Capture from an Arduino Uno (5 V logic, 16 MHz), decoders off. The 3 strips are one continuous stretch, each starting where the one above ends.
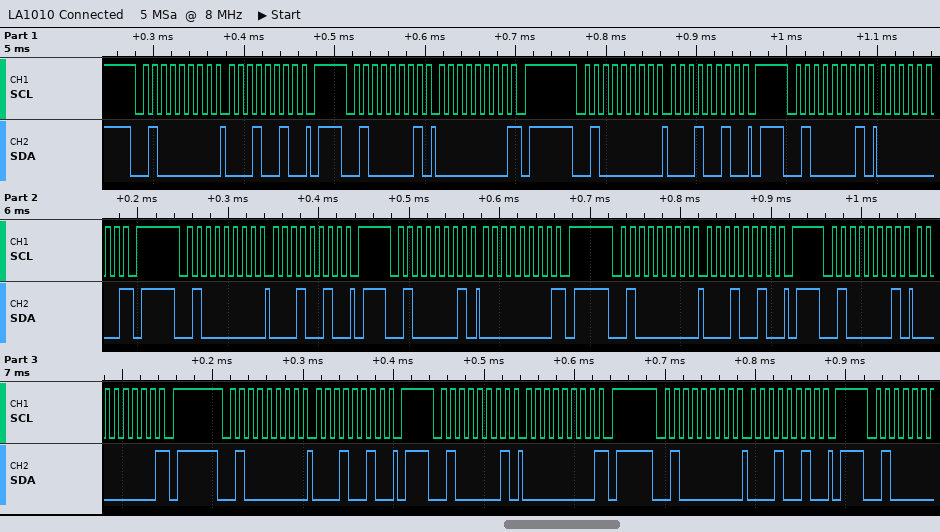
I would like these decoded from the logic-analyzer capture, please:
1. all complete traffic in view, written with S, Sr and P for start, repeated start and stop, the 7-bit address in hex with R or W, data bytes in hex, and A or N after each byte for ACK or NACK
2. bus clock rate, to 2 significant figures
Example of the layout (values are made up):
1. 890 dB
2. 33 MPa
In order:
1. S 20W A 12 A P S 20R A 00 N P S 20W A 12 A P S 20R A 00 N P S 20W A 12 A P S 20R A 00 N P S 20W A 12 A P S 20R A 00 N P S 20W A 12 A P S 20R A 00 N P S 20W A 12 A P
2. 100 kHz
